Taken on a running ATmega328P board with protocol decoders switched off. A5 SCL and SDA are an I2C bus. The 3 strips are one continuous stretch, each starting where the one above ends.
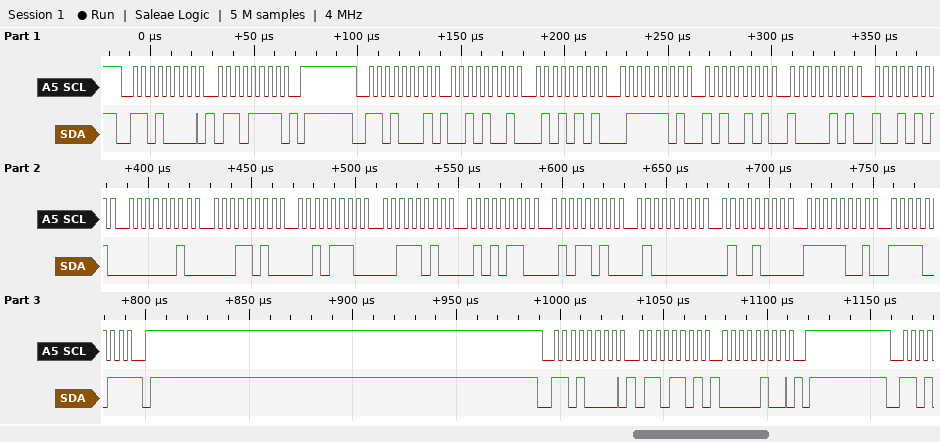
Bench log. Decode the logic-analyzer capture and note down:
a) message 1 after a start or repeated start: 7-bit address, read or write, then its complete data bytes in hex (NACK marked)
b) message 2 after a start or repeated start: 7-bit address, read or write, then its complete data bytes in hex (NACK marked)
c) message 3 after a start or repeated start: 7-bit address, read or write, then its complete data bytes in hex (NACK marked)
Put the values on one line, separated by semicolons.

0x68 write: 6F; 0x68 read: 29 55 7D A5 85 95 02 1A 2E 3A 56 5A 40 48 F9 F3 NACK; 0x68 write: 6D 04
